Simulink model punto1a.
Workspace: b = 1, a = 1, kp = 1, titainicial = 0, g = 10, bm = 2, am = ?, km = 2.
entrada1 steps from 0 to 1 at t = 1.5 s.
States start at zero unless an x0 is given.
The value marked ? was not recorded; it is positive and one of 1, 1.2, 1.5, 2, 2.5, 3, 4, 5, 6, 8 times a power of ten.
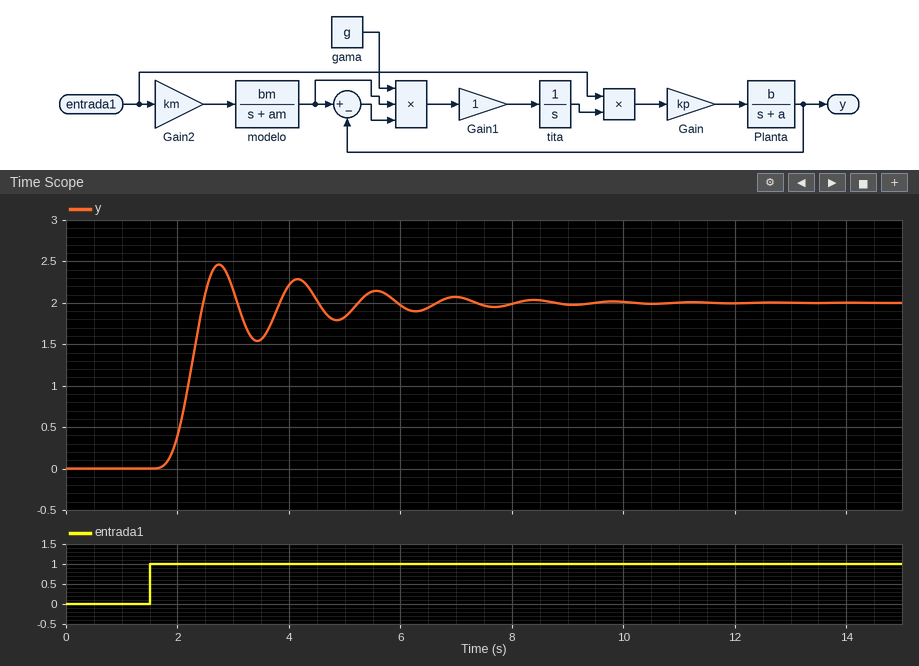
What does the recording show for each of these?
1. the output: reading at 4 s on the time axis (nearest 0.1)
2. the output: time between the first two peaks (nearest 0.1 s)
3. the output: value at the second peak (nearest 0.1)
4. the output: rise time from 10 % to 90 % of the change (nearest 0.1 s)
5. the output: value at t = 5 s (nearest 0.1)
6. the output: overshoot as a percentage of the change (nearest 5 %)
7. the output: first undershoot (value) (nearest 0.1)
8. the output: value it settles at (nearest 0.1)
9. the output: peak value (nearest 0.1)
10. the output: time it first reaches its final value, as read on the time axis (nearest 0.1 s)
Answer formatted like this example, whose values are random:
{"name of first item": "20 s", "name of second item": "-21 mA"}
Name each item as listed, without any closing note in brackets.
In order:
{"the output: reading at 4 s on the time axis": "2.2", "the output: time between the first two peaks": "1.4 s", "the output: value at the second peak": "2.3", "the output: rise time from 10 % to 90 % of the change": "0.5 s", "the output: value at t = 5 s": "1.8", "the output: overshoot as a percentage of the change": "25 %", "the output: first undershoot (value)": "1.5", "the output: value it settles at": "2.0", "the output: peak value": "2.5", "the output: time it first reaches its final value, as read on the time axis": "2.5 s"}
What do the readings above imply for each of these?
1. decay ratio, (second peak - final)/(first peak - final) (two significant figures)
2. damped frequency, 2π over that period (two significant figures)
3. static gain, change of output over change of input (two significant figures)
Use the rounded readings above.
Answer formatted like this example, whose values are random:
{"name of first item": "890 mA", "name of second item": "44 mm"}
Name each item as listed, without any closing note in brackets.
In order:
{"decay ratio, (second peak - final)/(first peak - final)": "0.60", "damped frequency, 2π over that period": "4.5 rad/s", "static gain, change of output over change of input": "2.0"}
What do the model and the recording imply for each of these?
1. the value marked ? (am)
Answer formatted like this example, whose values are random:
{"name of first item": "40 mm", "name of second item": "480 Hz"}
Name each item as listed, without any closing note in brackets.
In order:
{"the value marked ?": "2"}
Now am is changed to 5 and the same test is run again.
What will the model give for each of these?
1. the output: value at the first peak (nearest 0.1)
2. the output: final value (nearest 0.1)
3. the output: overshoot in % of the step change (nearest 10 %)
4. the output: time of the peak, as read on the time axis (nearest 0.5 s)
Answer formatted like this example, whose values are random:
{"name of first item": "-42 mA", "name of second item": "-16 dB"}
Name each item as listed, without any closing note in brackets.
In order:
{"the output: value at the first peak": "1.2", "the output: final value": "0.8", "the output: overshoot in % of the step change": "50 %", "the output: time of the peak, as read on the time axis": "3.0 s"}
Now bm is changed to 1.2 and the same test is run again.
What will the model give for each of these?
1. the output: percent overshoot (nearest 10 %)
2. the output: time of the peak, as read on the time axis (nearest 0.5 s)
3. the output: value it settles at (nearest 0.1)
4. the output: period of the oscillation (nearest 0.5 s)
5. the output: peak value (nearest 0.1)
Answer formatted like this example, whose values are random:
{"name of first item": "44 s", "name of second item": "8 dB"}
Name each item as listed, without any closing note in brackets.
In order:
{"the output: percent overshoot": "30 %", "the output: time of the peak, as read on the time axis": "3.0 s", "the output: value it settles at": "1.2", "the output: period of the oscillation": "2.0 s", "the output: peak value": "1.5"}
